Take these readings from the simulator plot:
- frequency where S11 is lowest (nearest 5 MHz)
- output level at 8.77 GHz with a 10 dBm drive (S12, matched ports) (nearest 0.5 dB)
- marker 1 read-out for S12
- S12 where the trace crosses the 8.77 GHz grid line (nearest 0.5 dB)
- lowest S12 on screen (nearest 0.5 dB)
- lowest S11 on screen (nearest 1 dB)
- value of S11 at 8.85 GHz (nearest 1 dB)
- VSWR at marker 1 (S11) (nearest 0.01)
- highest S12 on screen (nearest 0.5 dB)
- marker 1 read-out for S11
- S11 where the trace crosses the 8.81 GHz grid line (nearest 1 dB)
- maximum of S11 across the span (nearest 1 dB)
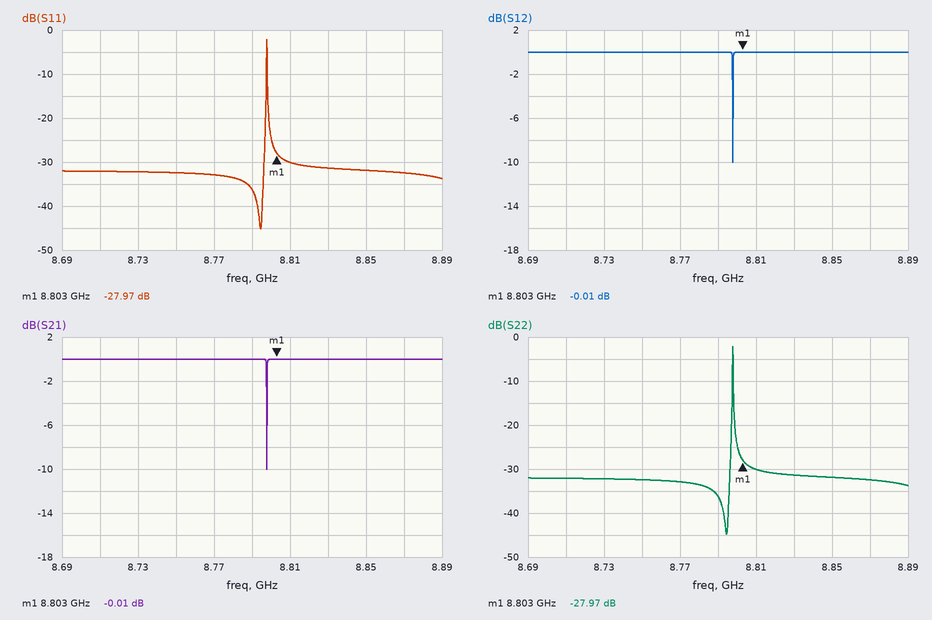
8.795 GHz
10.0 dBm
-0.01 dB
0.0 dB
-10.0 dB
-45 dB
-32 dB
1.08
0.0 dB
-27.97 dB
-30 dB
-2 dB
